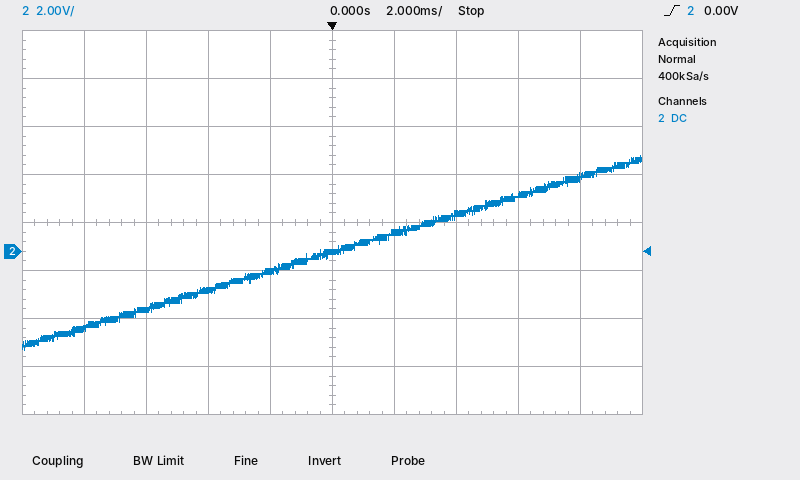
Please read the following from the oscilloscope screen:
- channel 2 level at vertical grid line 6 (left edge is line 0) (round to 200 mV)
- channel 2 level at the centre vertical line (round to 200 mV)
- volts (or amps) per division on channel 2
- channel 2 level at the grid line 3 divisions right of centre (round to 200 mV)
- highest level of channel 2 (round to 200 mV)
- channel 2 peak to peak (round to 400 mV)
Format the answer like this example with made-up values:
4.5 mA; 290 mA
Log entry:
800 mV; 0.0 V; 2 V; 2.4 V; 4.0 V; 8.0 V
